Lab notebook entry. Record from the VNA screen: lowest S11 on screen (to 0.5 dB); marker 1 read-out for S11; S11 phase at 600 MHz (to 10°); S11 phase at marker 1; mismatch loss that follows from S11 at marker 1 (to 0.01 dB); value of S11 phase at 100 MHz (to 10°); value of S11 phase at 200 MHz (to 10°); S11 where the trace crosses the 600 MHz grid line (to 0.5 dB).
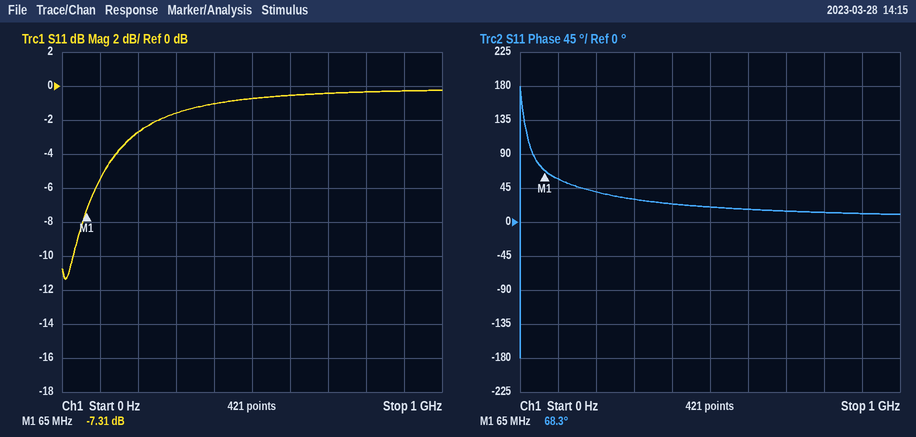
-11.5 dB
-7.31 dB
20°
68.3°
0.89 dB
60°
40°
-0.5 dB
